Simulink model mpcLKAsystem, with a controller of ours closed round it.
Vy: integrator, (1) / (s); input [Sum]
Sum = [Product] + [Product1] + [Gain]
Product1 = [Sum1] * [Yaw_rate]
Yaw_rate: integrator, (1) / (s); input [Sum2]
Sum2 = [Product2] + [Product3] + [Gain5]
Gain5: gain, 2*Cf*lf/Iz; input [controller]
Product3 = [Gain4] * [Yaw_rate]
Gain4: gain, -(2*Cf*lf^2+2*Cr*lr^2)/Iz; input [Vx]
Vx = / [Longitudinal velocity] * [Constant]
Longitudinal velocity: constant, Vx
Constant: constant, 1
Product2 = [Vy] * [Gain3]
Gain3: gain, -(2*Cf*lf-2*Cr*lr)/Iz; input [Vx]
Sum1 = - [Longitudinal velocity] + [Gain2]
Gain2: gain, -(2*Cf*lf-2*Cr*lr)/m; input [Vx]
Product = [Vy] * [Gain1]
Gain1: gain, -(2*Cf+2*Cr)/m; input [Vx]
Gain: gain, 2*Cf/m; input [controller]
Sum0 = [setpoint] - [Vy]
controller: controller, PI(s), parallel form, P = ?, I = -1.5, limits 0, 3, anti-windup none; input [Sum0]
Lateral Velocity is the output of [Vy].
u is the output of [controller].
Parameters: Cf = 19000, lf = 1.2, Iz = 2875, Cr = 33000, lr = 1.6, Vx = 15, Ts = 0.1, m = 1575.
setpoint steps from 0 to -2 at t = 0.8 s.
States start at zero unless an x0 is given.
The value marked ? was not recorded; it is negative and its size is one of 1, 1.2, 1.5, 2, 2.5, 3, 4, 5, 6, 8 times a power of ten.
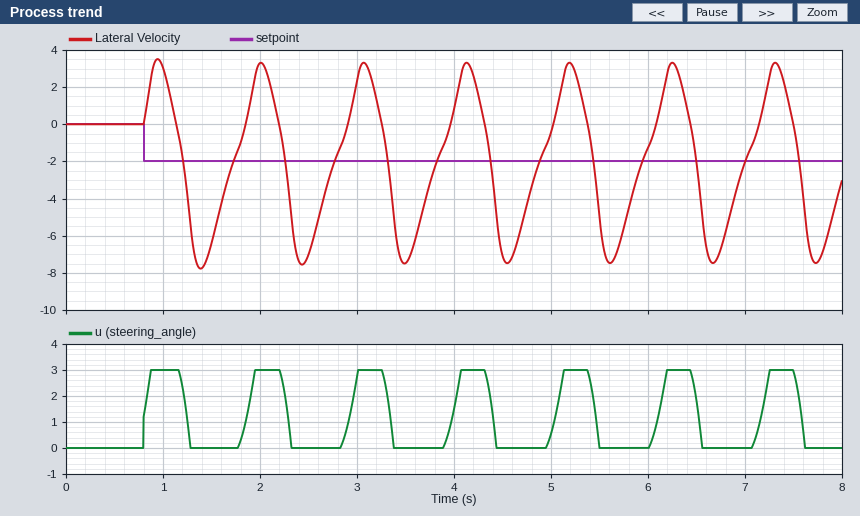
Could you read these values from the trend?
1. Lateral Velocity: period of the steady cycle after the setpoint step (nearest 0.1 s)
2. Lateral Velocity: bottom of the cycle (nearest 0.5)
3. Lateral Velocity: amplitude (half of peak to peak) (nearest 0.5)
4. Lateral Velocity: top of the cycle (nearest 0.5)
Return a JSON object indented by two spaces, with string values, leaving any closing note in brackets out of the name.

{
  "Lateral Velocity: period of the steady cycle after the setpoint step": "1.1 s",
  "Lateral Velocity: bottom of the cycle": "-7.5",
  "Lateral Velocity: amplitude (half of peak to peak)": "5.5",
  "Lateral Velocity: top of the cycle": "3.5"
}
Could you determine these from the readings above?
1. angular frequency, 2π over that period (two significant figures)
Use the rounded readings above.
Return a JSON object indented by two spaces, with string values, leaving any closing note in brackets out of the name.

{
  "angular frequency, 2π over that period": "5.7 rad/s"
}
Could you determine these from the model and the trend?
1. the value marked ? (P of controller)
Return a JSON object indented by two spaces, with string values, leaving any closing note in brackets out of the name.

{
  "the value marked ?": "-0.6"
}
